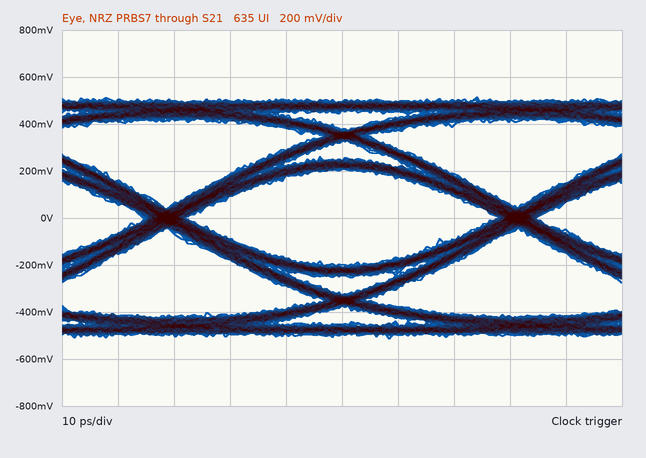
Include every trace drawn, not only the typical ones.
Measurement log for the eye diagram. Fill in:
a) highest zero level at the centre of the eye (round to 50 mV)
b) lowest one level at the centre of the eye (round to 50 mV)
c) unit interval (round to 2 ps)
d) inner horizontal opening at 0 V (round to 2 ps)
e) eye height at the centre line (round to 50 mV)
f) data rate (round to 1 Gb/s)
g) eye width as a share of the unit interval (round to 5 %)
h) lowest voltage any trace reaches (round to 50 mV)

-200 mV
200 mV
62 ps
56 ps
400 mV
16 Gb/s
90 %
-500 mV
